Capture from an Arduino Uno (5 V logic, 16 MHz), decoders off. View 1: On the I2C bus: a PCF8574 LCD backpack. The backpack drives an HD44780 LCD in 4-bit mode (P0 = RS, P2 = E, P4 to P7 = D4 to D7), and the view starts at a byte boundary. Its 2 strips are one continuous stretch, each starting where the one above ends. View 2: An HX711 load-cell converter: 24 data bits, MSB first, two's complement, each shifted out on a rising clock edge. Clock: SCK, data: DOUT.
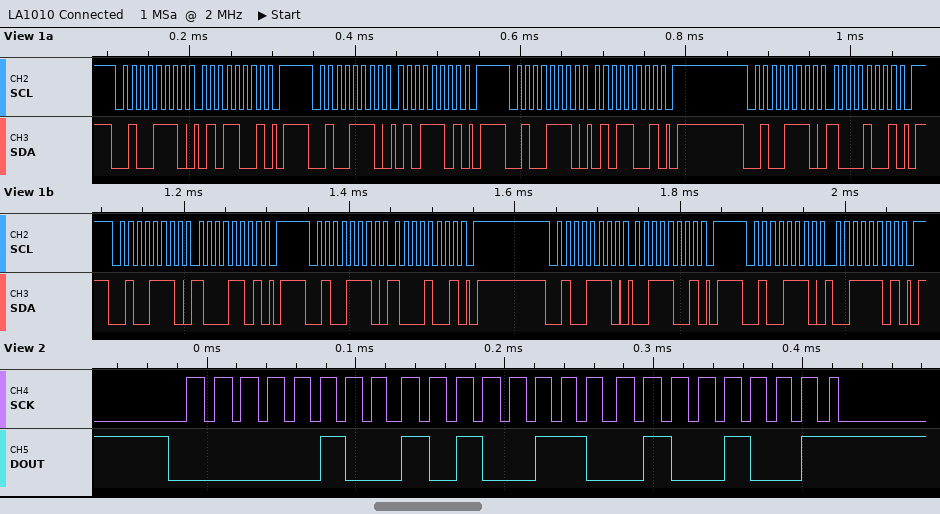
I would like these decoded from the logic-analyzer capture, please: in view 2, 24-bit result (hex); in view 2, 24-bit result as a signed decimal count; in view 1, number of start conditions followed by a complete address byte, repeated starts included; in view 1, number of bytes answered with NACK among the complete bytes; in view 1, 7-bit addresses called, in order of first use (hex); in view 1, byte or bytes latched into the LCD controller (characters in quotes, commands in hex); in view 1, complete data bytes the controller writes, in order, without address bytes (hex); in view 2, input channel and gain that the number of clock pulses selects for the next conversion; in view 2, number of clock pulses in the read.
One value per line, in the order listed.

0x04A649
304713
8
0
0x27
'X'
59 5D 59 89 8D 89 39 3D
channel A, gain 128
25
